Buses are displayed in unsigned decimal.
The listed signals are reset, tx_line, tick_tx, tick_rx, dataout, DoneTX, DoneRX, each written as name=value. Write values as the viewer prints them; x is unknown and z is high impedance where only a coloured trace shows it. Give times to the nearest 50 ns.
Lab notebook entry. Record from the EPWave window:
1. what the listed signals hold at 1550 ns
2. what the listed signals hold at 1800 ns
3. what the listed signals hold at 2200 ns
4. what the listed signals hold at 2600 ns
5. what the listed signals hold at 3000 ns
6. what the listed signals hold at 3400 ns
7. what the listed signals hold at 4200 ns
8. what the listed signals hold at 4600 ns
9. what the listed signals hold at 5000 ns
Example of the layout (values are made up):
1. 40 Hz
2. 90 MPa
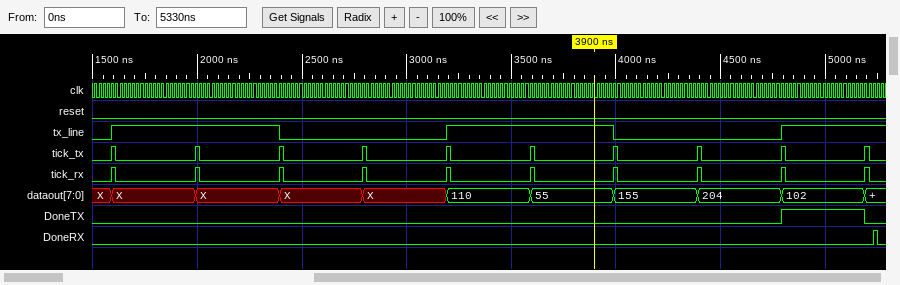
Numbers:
1. reset=0, tx_line=0, tick_tx=0, tick_rx=0, dataout=X, DoneTX=0, DoneRX=0
2. reset=0, tx_line=1, tick_tx=0, tick_rx=0, dataout=X, DoneTX=0, DoneRX=0
3. reset=0, tx_line=1, tick_tx=0, tick_rx=0, dataout=X, DoneTX=0, DoneRX=0
4. reset=0, tx_line=0, tick_tx=0, tick_rx=0, dataout=X, DoneTX=0, DoneRX=0
5. reset=0, tx_line=0, tick_tx=0, tick_rx=0, dataout=X, DoneTX=0, DoneRX=0
6. reset=0, tx_line=1, tick_tx=0, tick_rx=0, dataout=110, DoneTX=0, DoneRX=0
7. reset=0, tx_line=0, tick_tx=0, tick_rx=0, dataout=155, DoneTX=0, DoneRX=0
8. reset=0, tx_line=0, tick_tx=0, tick_rx=0, dataout=204, DoneTX=0, DoneRX=0
9. reset=0, tx_line=1, tick_tx=0, tick_rx=0, dataout=102, DoneTX=1, DoneRX=0
